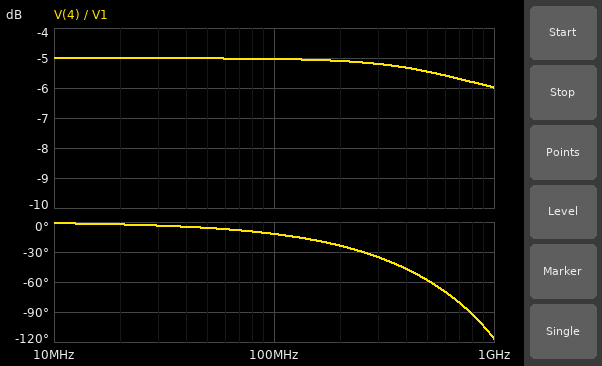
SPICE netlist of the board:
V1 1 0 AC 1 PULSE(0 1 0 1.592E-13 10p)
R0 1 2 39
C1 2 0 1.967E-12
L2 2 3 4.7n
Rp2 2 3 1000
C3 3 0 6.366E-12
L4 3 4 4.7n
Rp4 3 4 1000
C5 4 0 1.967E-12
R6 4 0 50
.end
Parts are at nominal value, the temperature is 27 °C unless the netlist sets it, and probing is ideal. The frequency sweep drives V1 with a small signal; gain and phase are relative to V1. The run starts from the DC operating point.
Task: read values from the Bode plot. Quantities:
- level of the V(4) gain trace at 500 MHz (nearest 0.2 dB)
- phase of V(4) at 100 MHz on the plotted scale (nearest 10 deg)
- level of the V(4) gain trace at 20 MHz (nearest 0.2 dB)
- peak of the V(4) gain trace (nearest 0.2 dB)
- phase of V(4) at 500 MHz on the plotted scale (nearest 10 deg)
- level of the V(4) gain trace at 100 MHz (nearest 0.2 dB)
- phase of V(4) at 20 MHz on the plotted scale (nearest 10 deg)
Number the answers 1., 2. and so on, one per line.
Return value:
1. -5.4 dB
2. -10 deg
3. -5.0 dB
4. -5.0 dB
5. -60 deg
6. -5.0 dB
7. 0 deg
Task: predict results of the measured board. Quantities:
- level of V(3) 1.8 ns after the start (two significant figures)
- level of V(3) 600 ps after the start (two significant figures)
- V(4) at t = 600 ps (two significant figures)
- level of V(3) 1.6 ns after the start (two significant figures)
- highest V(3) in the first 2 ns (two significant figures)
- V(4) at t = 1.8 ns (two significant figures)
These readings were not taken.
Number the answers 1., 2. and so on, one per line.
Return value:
1. 560 mV
2. 530 mV
3. 600 mV
4. 560 mV
5. 570 mV
6. 560 mV
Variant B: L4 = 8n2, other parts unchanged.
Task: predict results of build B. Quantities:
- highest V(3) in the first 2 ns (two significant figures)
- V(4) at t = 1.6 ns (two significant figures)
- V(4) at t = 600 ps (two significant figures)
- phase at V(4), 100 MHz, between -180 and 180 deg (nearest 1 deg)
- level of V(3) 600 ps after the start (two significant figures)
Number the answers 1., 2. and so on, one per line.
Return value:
1. 620 mV
2. 560 mV
3. 570 mV
4. -13 deg
5. 560 mV
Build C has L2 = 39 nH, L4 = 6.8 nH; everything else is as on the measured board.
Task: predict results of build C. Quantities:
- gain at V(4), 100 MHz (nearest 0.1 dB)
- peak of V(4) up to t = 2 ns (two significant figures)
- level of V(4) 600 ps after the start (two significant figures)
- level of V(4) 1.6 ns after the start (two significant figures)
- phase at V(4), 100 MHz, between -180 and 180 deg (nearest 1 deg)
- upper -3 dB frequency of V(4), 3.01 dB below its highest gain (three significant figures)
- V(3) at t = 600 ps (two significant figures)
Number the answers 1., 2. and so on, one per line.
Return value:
1. -5.2 dB
2. 570 mV
3. 220 mV
4. 550 mV
5. -27 deg
6. 379 MHz
7. 310 mV
